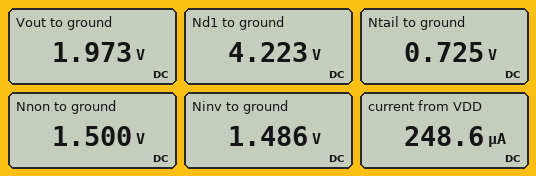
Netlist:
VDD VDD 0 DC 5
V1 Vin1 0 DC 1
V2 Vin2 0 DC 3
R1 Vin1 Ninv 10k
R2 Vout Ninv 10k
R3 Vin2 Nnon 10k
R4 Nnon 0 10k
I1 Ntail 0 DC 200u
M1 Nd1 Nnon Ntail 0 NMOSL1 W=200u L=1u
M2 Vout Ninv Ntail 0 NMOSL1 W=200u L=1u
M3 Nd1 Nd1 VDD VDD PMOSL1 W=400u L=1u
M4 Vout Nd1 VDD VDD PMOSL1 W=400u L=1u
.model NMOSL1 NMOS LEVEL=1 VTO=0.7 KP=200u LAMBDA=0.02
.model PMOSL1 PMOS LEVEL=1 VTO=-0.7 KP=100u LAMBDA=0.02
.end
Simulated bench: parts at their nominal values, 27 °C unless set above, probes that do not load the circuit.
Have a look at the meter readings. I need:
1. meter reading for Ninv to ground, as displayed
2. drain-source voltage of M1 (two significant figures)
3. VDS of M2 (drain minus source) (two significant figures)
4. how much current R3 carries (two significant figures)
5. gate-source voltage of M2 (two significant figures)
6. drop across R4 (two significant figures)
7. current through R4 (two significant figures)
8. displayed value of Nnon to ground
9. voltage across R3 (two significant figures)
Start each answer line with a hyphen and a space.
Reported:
- 1.486 V
- 3.5 V
- 1.2 V
- 150 µA
- 760 mV
- 1.5 V
- 150 µA
- 1.500 V
- 1.5 V
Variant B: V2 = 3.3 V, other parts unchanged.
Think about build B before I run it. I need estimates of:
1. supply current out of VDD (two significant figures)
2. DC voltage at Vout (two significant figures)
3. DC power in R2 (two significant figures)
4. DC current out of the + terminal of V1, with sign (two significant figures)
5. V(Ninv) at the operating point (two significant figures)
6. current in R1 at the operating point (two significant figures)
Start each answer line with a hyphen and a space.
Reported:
- 260 µA
- 2.3 V
- 40 µW
- -63 µA
- 1.6 V
- 63 µA
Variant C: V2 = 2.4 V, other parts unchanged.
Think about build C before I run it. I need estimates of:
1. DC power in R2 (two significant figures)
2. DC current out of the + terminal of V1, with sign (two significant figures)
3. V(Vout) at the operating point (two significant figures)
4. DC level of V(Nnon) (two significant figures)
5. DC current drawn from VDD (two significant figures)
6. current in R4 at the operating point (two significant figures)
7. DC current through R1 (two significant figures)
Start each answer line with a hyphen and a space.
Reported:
- 3.9 µW
- -20 µA
- 1.4 V
- 1.2 V
- 220 µA
- 120 µA
- 20 µA
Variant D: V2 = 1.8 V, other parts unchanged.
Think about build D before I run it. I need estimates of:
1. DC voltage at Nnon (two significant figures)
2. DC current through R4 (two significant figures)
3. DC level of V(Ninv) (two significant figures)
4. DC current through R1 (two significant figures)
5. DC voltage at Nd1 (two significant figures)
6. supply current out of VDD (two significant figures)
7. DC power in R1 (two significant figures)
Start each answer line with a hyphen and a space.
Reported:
- 900 mV
- 90 µA
- 910 mV
- 9.2 µA
- 4.2 V
- 190 µA
- 850 nW
